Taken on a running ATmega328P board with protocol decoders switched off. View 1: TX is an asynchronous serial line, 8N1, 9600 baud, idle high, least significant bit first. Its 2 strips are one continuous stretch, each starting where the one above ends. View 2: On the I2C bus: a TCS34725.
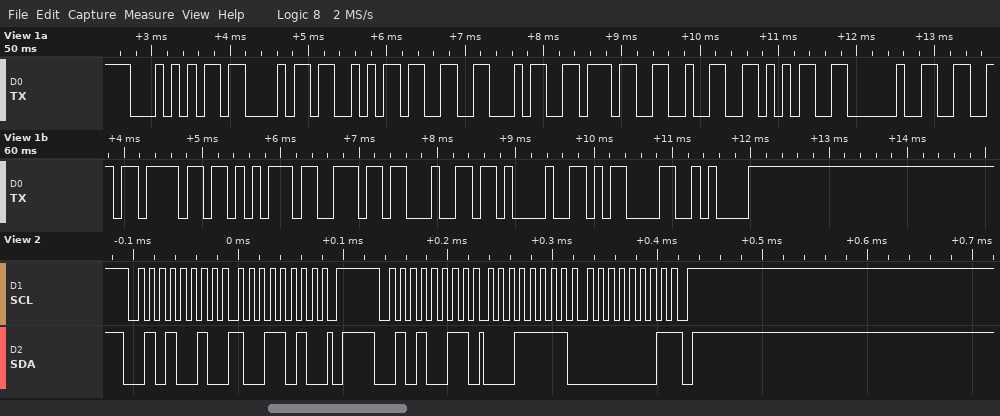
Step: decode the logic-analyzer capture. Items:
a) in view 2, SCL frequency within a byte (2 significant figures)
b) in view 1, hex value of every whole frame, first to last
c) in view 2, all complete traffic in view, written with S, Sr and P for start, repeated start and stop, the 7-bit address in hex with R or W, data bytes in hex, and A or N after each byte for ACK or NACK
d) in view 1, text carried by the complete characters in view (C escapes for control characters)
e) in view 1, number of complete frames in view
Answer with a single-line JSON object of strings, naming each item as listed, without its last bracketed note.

{"in view 2, SCL frequency within a byte": "100 kHz", "in view 1, hex value of every whole frame, first to last": "54 43 53 33 34 37 32 35 20 66 6F 75 6E 64 21 0D 0A", "in view 2, all complete traffic in view, written with S, Sr and P for start, repeated start and stop, the 7-bit address in hex with R or W, data bytes in hex, and A or N after each byte for ACK or NACK": "S 29W A 9A A P S 29R A 1F A 01 N P", "in view 1, text carried by the complete characters in view": "\"TCS34725 found!\\r\\n\"", "in view 1, number of complete frames in view": "17"}
